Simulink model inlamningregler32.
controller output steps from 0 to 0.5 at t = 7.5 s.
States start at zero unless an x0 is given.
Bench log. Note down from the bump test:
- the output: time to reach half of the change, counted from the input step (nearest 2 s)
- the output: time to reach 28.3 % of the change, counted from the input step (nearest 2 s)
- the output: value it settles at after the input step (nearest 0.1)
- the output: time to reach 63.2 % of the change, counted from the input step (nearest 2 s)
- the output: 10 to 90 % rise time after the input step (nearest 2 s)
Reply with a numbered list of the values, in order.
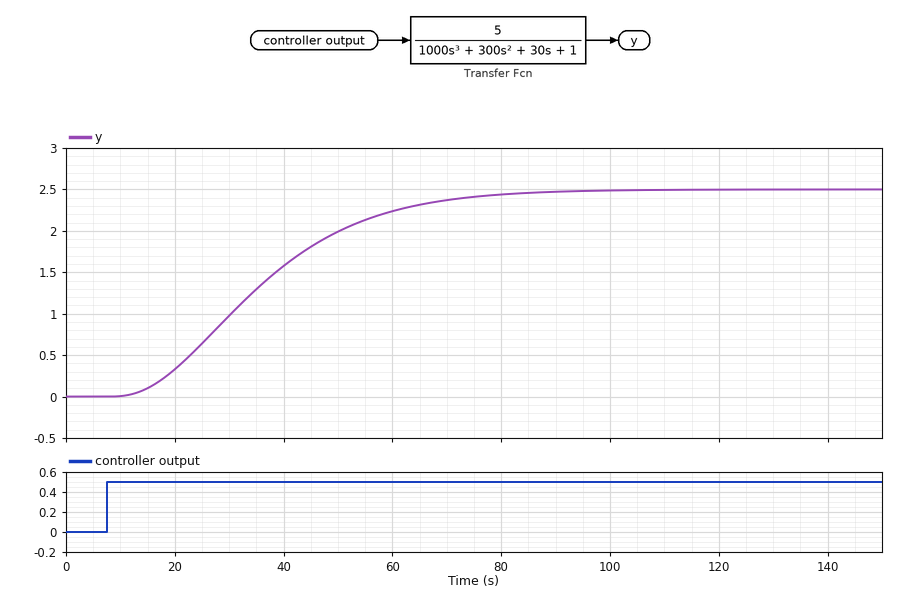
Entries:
1. 26 s
2. 18 s
3. 2.5
4. 32 s
5. 42 s
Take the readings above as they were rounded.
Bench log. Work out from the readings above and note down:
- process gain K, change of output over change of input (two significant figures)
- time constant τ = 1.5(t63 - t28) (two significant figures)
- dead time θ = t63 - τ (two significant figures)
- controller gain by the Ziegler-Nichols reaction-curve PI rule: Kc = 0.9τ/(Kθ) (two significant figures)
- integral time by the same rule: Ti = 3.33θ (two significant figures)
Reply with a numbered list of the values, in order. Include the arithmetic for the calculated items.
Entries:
1. (2.5 - 0) / 0.5 = 5.0
2. 1.5 × (32 - 18) = 21 s
3. 32 - 21 = 11 s
4. 0.9 × 21 / (5 × 11) = 0.34
5. 3.33 × 11 = 37 s
